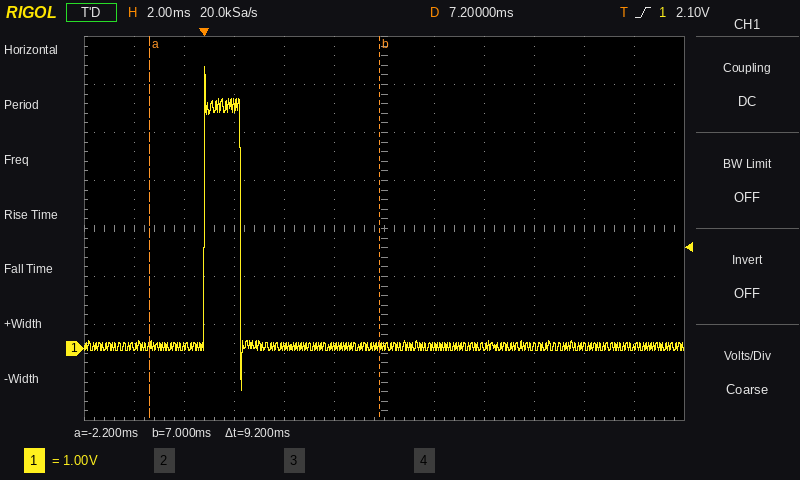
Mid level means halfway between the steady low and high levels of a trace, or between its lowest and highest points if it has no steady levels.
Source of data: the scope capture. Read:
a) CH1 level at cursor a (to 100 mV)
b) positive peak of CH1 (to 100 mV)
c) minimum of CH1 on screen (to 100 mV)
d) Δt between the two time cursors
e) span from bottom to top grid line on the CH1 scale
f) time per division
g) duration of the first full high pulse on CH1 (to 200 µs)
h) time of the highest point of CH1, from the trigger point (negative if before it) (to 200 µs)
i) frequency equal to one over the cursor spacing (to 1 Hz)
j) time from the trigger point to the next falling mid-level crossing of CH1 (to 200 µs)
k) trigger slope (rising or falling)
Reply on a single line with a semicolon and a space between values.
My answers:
100 mV; 5.9 V; -900 mV; 9.2 ms; 8 V; 2 ms; 1.4 ms; 0.0 ms; 109 Hz; 1.4 ms; rising
